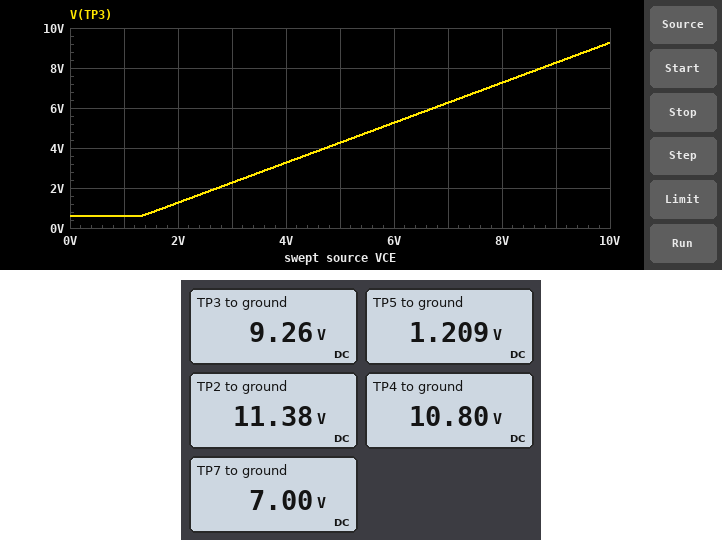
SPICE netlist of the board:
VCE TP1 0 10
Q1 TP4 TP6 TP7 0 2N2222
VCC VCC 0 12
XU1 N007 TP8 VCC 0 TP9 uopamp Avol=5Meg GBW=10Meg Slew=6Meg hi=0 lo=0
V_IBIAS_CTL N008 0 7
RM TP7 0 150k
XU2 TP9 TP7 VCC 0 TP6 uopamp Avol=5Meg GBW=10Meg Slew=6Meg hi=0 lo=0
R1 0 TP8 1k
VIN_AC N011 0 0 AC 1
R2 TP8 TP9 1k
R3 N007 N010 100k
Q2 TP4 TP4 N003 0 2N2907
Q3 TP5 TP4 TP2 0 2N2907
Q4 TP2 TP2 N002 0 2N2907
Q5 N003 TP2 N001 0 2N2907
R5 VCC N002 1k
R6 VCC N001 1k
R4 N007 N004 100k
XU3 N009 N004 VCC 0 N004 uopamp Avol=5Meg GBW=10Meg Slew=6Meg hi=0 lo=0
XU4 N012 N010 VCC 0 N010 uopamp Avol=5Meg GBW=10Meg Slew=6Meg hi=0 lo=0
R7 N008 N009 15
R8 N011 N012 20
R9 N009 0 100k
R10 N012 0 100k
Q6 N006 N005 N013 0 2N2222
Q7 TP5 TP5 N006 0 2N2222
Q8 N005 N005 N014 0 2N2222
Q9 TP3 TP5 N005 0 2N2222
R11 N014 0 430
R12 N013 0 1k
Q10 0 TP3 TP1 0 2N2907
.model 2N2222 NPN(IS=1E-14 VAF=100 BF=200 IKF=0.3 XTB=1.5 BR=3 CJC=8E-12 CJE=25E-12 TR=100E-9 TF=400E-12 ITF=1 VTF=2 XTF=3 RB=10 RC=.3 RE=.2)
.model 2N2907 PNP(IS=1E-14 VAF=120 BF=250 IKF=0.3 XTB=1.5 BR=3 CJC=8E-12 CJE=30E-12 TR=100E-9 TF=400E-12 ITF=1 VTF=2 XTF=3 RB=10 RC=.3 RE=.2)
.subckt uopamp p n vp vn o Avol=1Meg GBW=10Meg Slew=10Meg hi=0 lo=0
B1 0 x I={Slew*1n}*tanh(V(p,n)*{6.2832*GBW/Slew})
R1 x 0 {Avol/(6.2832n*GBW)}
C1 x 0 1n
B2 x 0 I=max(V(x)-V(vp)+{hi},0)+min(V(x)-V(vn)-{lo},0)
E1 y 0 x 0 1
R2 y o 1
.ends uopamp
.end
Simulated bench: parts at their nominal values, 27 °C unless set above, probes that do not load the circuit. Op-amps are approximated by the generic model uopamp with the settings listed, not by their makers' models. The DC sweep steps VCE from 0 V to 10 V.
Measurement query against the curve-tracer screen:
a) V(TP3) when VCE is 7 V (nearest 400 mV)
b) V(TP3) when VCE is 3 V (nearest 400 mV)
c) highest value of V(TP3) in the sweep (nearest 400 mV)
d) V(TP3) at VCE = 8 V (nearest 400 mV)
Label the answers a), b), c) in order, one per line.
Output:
a) 6.4 V
b) 2.4 V
c) 9.2 V
d) 7.2 V
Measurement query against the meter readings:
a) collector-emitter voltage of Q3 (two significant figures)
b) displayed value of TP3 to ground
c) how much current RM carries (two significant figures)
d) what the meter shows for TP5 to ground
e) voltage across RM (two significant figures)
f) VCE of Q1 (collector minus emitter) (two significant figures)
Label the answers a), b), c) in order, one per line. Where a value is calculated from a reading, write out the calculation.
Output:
a) 1.209 V - 11.38 V = -10 V
b) 9.26 V
c) (7 V) / 150 kΩ = 47 µA
d) 1.209 V
e) 7 V = 7.0 V
f) 10.8 V - 7 V = 3.8 V
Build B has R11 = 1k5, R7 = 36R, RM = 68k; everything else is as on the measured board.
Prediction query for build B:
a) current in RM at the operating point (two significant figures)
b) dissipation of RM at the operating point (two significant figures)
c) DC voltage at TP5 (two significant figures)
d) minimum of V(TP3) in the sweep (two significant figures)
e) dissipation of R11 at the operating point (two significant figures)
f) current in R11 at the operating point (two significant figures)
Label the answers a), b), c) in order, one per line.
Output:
a) 100 µA
b) 720 µW
c) 1.3 V
d) 650 mV
e) 8.2 µW
f) 74 µA
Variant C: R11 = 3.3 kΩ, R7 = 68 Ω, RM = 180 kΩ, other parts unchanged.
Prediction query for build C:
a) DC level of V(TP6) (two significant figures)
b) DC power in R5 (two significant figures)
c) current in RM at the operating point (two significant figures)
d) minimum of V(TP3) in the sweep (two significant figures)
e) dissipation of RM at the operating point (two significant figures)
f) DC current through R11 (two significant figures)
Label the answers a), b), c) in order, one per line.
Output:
a) 7.6 V
b) 1.5 µW
c) 39 µA
d) 590 mV
e) 270 µW
f) 18 µA
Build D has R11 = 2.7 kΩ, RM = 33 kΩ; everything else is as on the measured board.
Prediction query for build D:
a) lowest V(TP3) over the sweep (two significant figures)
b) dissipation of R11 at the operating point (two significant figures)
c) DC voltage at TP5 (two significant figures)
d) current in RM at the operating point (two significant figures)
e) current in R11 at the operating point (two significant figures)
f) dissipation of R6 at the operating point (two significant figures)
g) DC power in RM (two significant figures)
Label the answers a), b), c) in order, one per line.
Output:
a) 760 mV
b) 20 µW
c) 1.4 V
d) 210 µA
e) 87 µA
f) 45 µW
g) 1.5 mW
